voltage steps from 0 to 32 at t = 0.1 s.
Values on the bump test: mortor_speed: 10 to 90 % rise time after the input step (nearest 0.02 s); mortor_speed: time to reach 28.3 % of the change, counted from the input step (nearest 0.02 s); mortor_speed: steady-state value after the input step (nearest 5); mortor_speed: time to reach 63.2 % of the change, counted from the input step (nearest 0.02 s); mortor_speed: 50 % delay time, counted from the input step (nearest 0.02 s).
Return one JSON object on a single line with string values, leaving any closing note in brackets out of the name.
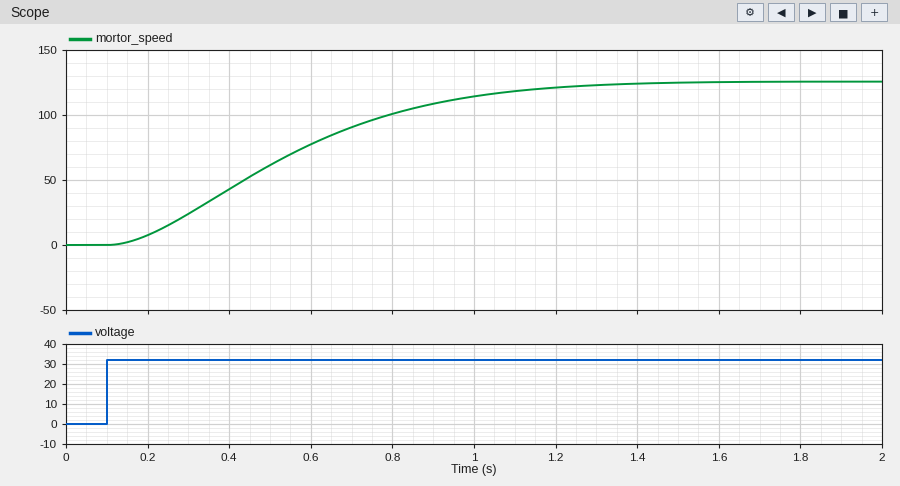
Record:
{"mortor_speed: 10 to 90 % rise time after the input step": "0.74 s", "mortor_speed: time to reach 28.3 % of the change, counted from the input step": "0.26 s", "mortor_speed: steady-state value after the input step": "125", "mortor_speed: time to reach 63.2 % of the change, counted from the input step": "0.52 s", "mortor_speed: 50 % delay time, counted from the input step": "0.40 s"}
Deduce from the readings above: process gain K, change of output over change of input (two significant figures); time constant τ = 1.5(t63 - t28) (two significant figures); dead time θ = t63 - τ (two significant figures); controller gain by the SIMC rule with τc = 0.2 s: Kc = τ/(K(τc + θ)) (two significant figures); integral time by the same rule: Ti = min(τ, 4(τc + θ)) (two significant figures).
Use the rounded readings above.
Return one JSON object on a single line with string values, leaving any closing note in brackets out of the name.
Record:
{"process gain K, change of output over change of input": "3.9", "time constant τ = 1.5(t63 - t28)": "0.39 s", "dead time θ = t63 - τ": "0.13 s", "controller gain by the SIMC rule with τc = 0.2 s: Kc = τ/(K(τc + θ))": "0.30", "integral time by the same rule: Ti = min(τ, 4(τc + θ))": "0.39 s"}
